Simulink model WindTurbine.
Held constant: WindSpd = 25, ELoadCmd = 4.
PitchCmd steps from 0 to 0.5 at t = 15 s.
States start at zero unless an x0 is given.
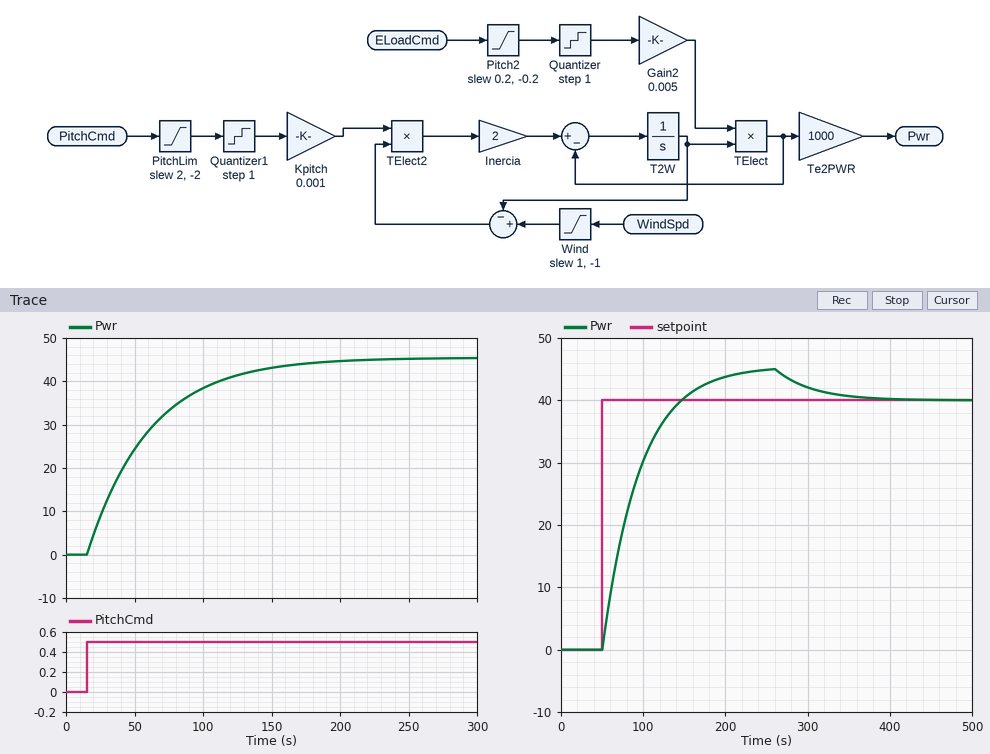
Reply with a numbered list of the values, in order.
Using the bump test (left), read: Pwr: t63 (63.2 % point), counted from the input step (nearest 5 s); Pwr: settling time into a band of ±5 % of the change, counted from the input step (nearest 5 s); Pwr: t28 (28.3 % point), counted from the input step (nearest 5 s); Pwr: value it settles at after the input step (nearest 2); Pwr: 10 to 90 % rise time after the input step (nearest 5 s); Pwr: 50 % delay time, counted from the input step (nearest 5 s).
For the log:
1. 45 s
2. 135 s
3. 15 s
4. 46
5. 100 s
6. 30 s
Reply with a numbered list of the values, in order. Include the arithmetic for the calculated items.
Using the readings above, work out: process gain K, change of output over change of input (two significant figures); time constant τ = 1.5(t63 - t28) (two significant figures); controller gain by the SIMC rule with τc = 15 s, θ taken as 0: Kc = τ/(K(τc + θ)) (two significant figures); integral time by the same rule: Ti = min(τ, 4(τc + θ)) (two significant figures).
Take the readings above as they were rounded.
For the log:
1. (46 - 0) / 0.5 = 92
2. 1.5 × (45 - 15) = 45 s
3. 45 / (92 × (15 + 0)) = 0.033
4. min(45, 4 × (15 + 0)) = 45 s
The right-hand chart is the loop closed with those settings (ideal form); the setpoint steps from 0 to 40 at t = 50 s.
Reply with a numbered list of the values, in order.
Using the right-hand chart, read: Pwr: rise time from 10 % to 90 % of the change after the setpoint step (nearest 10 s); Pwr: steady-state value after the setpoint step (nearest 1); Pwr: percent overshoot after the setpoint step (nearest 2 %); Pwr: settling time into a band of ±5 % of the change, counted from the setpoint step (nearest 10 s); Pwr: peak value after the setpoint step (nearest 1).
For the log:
1. 70 s
2. 40
3. 12 %
4. 250 s
5. 45
